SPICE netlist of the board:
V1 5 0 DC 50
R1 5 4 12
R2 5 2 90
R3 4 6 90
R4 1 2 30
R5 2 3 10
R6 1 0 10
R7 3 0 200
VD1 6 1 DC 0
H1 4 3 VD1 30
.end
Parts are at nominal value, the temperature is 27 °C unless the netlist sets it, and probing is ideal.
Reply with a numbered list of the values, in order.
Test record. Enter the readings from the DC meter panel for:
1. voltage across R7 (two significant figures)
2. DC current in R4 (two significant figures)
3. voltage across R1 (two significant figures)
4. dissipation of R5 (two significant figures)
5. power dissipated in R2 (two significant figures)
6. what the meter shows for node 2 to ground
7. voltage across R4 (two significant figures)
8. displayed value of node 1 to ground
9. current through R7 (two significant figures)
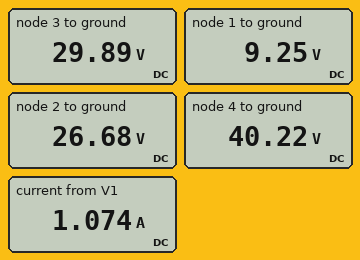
1. 30 V
2. 580 mA
3. 9.8 V
4. 1.0 W
5. 6.0 W
6. 26.68 V
7. 17 V
8. 9.25 V
9. 150 mA
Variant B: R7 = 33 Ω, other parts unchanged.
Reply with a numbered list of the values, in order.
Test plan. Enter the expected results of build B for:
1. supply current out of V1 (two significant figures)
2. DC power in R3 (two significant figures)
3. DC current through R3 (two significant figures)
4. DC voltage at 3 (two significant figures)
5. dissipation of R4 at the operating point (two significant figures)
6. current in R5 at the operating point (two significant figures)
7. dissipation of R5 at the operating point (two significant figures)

1. 1.6 A
2. 7.8 W
3. 290 mA
4. 26 V
5. 7.9 W
6. 220 mA
7. 480 mW
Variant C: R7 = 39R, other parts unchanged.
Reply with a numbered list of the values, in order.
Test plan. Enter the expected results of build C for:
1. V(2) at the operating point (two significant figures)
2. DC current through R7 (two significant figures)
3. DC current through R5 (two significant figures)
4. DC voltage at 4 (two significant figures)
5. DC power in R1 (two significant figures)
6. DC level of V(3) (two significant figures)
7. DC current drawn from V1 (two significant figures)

1. 24 V
2. 680 mA
3. 240 mA
4. 35 V
5. 18 W
6. 26 V
7. 1.5 A
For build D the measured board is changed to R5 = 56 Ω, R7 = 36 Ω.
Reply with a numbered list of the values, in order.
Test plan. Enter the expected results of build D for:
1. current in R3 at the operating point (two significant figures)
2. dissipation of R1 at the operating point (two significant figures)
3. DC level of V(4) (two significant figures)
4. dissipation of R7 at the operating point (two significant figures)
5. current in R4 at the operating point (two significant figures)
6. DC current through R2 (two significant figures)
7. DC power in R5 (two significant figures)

1. 320 mA
2. 16 W
3. 36 V
4. 20 W
5. 430 mA
6. 330 mA
7. 640 mW
